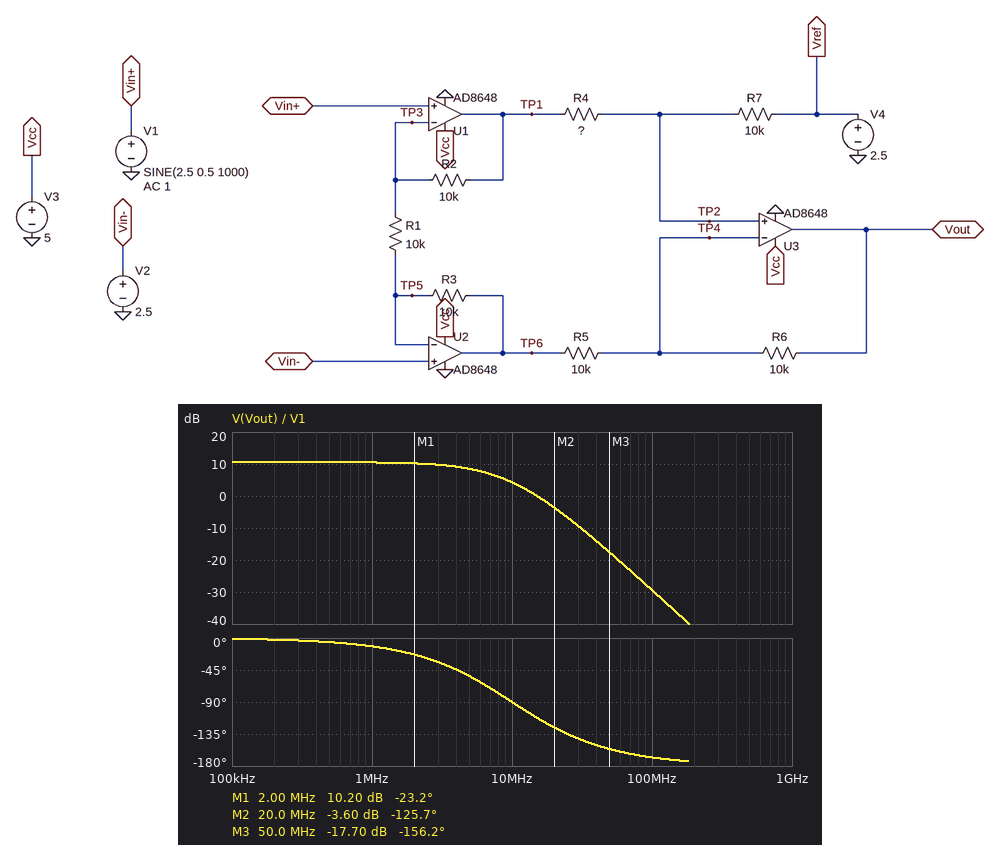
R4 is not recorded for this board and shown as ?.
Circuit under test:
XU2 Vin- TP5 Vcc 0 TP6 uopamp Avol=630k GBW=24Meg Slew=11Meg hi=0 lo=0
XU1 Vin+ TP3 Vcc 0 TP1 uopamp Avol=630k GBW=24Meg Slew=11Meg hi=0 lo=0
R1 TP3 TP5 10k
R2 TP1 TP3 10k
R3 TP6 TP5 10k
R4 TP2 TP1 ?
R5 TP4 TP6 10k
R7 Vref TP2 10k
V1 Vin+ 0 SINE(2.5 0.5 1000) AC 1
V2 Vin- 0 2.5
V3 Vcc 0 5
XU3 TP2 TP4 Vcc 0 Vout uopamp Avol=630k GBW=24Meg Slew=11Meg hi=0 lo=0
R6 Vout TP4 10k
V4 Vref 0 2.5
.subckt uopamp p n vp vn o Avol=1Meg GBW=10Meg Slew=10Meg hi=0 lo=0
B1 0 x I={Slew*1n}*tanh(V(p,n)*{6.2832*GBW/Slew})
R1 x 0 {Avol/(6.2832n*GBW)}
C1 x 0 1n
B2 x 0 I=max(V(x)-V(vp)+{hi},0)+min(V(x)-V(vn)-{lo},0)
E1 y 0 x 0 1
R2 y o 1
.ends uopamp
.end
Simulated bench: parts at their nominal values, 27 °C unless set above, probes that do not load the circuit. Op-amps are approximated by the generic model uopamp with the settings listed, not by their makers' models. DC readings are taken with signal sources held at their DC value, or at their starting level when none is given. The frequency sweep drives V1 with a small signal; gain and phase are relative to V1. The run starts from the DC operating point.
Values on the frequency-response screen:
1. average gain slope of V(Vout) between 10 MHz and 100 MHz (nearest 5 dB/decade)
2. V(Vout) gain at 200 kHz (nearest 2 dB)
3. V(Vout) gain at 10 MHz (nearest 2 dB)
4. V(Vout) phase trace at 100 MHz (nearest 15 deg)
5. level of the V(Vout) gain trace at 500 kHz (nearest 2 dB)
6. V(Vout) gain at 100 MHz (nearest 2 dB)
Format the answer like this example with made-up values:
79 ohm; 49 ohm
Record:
-35 dB/decade; 10 dB; 4 dB; -165 deg; 10 dB; -30 dB
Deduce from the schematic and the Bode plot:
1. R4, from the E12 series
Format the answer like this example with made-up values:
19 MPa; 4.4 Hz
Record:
6.8 kΩ
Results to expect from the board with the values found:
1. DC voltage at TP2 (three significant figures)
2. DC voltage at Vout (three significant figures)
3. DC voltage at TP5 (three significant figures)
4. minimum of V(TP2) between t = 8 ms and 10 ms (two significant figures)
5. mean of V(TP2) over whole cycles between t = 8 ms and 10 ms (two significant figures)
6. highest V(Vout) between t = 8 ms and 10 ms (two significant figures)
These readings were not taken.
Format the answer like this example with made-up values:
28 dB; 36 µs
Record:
2.50 V; 2.50 V; 2.50 V; 1.9 V; 2.5 V; 4.2 V
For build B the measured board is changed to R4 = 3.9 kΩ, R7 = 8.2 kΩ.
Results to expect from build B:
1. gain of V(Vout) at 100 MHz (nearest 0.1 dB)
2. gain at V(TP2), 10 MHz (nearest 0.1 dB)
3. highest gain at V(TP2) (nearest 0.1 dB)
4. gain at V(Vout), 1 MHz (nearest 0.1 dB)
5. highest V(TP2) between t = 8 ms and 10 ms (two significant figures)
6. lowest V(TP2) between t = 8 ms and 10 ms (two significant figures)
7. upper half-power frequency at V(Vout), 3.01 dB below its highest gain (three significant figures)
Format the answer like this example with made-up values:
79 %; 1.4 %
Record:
-28.3 dB; -0.7 dB; 2.6 dB; 11.3 dB; 3.2 V; 1.8 V; 6.19 MHz
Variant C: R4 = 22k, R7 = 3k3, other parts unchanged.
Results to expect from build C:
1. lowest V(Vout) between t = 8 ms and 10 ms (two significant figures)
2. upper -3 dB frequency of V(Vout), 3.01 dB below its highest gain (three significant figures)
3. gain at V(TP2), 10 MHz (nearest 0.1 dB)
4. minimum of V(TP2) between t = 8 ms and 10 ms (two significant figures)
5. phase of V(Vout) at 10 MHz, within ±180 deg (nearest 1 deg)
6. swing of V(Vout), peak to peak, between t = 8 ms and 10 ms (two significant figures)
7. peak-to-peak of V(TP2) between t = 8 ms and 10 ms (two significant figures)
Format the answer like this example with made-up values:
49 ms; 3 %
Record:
1.7 V; 5.90 MHz; -15.0 dB; 2.4 V; -102 deg; 1.5 V; 260 mV
